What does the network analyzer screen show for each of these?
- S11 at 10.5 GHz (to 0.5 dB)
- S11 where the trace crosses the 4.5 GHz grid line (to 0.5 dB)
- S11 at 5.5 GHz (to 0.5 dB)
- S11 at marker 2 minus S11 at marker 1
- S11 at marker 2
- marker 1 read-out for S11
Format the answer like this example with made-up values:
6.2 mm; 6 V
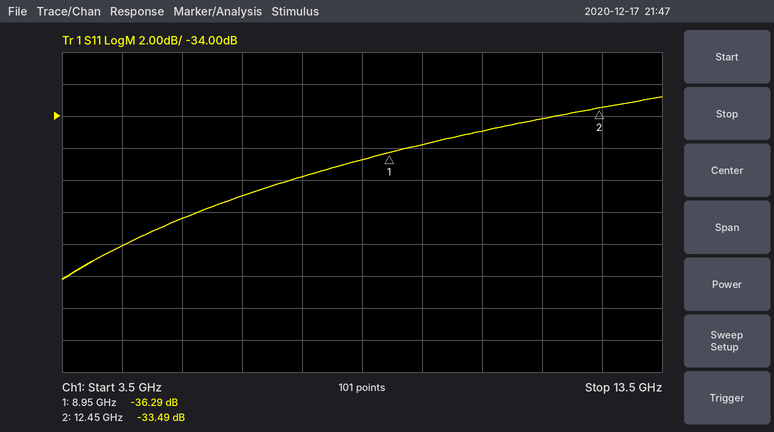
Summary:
-35.0 dB; -42.0 dB; -40.5 dB; 2.80 dB; -33.49 dB; -36.29 dB
